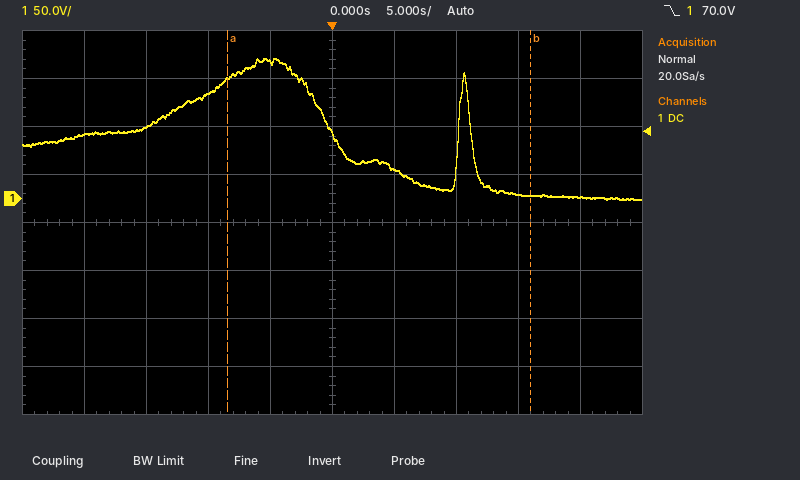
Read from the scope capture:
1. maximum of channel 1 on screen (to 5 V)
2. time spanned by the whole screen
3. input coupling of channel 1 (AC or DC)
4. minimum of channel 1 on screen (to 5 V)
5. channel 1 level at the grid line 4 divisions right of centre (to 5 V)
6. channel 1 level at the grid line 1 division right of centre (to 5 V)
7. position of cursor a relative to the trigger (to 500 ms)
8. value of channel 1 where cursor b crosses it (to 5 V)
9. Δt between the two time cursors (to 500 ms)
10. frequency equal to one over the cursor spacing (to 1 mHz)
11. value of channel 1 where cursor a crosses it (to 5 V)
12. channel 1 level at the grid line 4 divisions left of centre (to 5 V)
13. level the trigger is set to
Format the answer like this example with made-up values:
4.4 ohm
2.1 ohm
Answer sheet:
145 V
50 s
DC
0 V
0 V
30 V
-8.5 s
5 V
24.5 s
41 mHz
125 V
65 V
70.0 V
